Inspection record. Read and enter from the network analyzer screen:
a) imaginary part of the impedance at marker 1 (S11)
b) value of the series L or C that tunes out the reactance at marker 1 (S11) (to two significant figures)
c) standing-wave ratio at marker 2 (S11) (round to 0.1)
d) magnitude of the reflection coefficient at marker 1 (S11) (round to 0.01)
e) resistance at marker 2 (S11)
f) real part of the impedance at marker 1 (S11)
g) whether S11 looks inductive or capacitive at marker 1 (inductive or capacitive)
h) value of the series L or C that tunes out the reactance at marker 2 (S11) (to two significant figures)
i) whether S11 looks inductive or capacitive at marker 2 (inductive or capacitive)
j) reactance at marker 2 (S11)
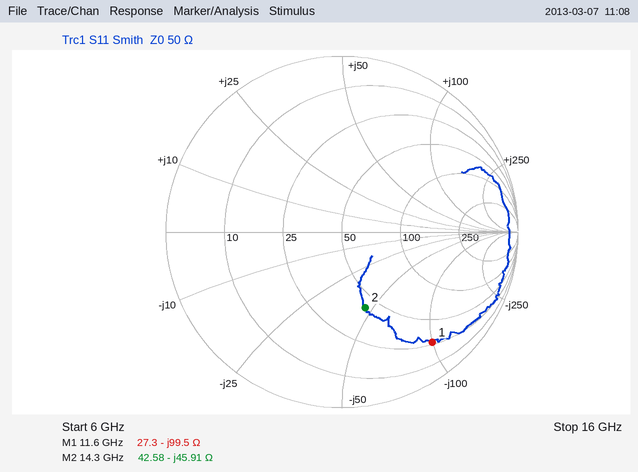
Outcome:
-99.5 Ω
1.4 nH
2.6
0.81
42.58 Ω
27.3 Ω
capacitive
510 pH
capacitive
-45.91 Ω
